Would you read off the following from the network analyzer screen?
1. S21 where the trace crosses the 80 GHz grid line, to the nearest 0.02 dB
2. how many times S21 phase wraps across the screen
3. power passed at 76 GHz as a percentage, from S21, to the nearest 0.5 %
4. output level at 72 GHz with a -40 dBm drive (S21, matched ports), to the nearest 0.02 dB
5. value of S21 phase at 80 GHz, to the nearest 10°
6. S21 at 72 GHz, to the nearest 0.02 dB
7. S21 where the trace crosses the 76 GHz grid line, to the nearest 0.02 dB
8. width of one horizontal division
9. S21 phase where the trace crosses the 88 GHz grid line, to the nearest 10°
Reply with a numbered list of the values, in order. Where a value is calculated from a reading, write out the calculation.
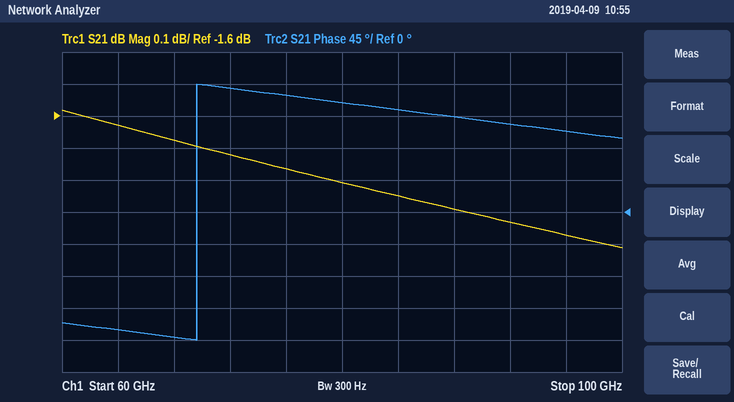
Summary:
1. -1.80 dB
2. 1
3. 10^(-1.76/10) ≈ 66.7 %, so 66.5 % to the nearest 0.5 %
4. -40 dBm + (-1.72 dB) = -41.72 dBm
5. 150°
6. -1.72 dB
7. -1.76 dB
8. 4 GHz
9. 130°
